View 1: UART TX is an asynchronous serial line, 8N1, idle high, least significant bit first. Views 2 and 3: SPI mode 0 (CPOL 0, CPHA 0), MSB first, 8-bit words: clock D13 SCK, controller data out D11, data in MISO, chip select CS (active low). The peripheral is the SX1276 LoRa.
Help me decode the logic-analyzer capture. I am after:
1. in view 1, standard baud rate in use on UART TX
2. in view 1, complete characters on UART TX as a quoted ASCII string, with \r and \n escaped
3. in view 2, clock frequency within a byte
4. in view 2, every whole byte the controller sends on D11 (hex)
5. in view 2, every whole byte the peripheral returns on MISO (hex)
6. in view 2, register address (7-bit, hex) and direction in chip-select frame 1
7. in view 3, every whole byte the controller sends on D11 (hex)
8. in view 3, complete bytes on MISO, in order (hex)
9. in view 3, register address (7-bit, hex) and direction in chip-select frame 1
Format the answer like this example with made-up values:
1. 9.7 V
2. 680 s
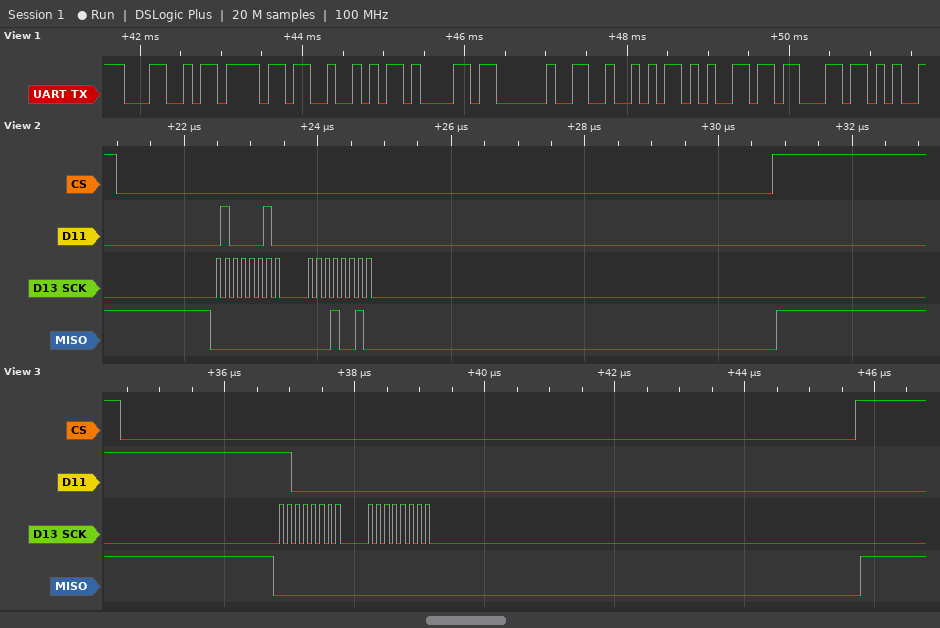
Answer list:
1. 9600 baud
2. "LoRa Rec"
3. 8 MHz
4. 42 00
5. 00 12
6. 0x42 read
7. C0 00
8. 00 00
9. 0x40 write
